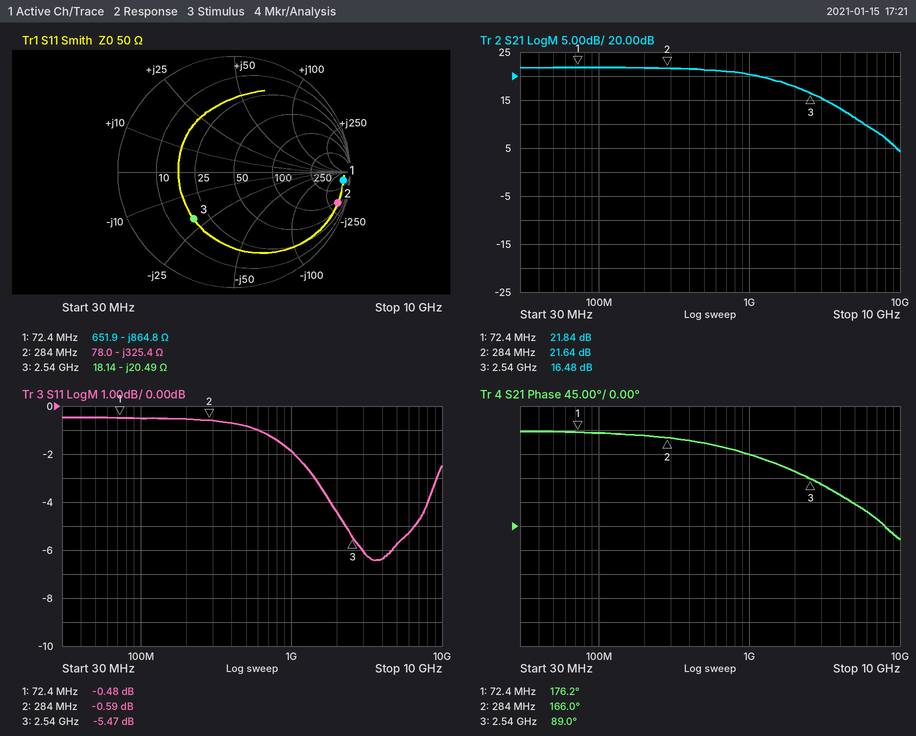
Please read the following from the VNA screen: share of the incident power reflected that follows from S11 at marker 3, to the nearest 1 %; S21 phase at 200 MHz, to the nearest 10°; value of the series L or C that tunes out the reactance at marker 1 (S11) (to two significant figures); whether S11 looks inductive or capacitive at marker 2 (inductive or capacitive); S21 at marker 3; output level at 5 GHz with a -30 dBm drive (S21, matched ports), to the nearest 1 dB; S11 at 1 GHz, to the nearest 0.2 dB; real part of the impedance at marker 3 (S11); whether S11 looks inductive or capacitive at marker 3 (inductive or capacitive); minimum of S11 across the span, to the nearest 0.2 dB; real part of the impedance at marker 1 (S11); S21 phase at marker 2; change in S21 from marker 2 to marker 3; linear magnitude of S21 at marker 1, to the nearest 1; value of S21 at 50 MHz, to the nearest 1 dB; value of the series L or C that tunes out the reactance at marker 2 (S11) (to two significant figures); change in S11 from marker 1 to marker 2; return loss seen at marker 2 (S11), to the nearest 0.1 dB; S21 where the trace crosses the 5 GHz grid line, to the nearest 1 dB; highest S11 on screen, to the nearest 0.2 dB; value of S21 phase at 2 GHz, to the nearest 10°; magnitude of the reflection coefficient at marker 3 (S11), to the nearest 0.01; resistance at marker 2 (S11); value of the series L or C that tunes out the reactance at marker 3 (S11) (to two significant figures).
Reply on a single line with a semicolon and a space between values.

28 %; 170°; 1.9 µH; capacitive; 16.48 dB; -19 dBm; -1.8 dB; 18.14 Ω; capacitive; -6.4 dB; 651.9 Ω; 166.0°; -5.16 dB; 12; 22 dB; 180 nH; -0.11 dB; 0.6 dB; 11 dB; -0.4 dB; 100°; 0.53; 78.0 Ω; 1.3 nH
